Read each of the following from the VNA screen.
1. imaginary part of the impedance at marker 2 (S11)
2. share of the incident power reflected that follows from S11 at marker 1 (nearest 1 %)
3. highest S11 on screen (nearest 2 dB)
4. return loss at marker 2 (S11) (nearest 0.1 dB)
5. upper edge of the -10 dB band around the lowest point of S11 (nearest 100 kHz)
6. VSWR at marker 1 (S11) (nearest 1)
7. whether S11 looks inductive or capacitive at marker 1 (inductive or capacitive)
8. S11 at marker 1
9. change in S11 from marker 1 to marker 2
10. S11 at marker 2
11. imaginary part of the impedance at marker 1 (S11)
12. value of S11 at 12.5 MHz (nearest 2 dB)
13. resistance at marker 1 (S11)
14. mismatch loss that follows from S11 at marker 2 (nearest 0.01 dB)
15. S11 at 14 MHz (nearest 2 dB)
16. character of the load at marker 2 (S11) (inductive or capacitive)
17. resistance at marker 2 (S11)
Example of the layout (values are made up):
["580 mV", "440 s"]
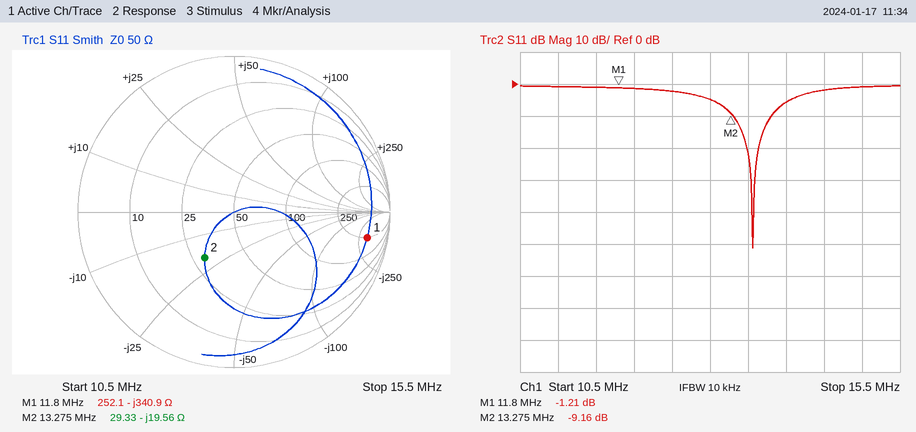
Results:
["-19.56 Ω", "76 %", "0 dB", "9.2 dB", "13.8 MHz", "14", "capacitive", "-1.21 dB", "-7.95 dB", "-9.16 dB", "-340.9 Ω", "-2 dB", "252.1 Ω", "0.56 dB", "-6 dB", "capacitive", "29.33 Ω"]
